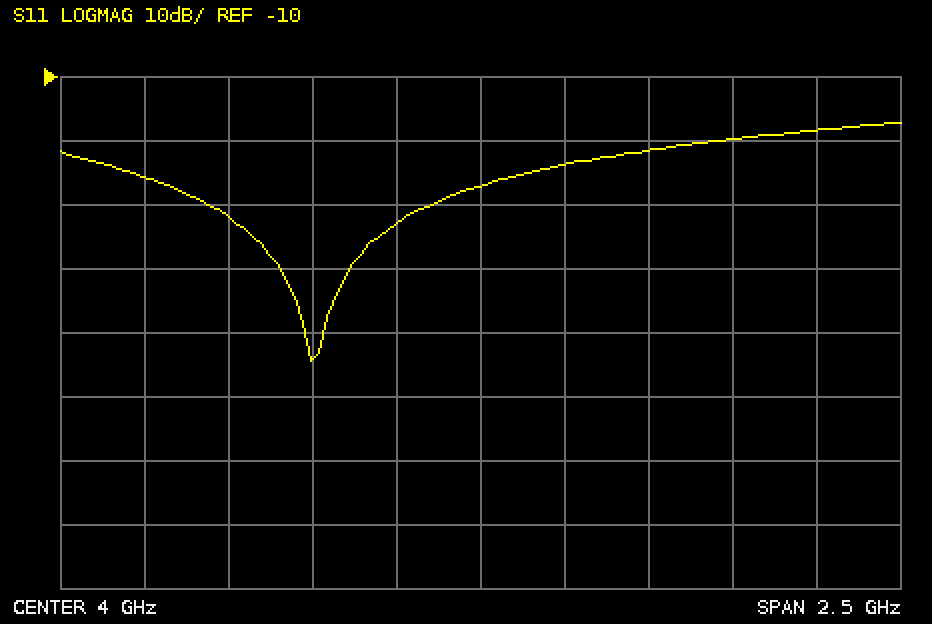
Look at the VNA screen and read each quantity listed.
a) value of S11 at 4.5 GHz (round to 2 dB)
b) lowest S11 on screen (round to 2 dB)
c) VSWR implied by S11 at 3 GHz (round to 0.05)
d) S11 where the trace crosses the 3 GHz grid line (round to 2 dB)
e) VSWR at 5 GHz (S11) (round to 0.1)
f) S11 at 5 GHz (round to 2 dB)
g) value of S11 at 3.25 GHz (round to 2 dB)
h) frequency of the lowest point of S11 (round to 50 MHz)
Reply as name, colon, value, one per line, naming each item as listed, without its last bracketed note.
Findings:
value of S11 at 4.5 GHz: -22 dB
lowest S11 on screen: -54 dB
VSWR implied by S11 at 3 GHz: 1.10
S11 where the trace crosses the 3 GHz grid line: -26 dB
VSWR at 5 GHz (S11): 1.3
S11 at 5 GHz: -18 dB
value of S11 at 3.25 GHz: -32 dB
frequency of the lowest point of S11: 3.50 GHz
